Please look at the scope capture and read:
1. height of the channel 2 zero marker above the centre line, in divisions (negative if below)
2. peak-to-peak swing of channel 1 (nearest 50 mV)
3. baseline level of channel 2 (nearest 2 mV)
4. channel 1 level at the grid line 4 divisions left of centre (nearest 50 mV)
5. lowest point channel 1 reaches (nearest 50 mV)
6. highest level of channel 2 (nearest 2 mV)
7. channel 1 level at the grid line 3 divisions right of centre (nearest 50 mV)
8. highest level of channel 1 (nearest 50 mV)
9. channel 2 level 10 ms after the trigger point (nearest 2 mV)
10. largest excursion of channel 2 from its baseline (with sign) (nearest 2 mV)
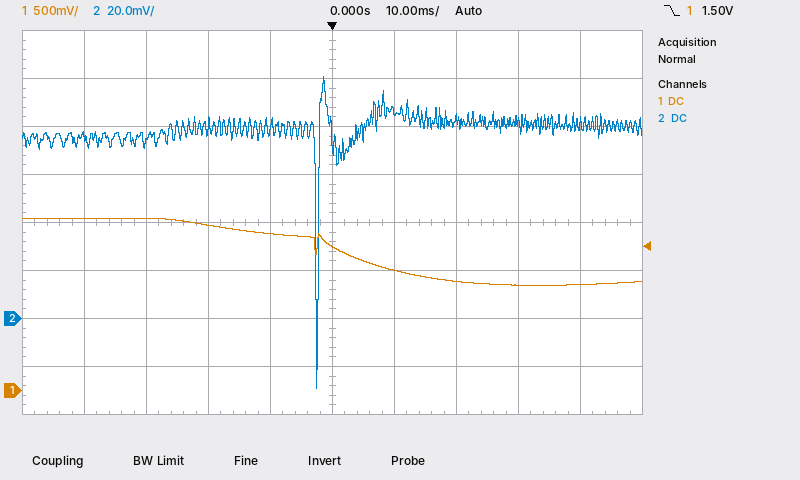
-2.0 div
700 mV
80 mV
1.80 V
1.10 V
100 mV
1.10 V
1.80 V
86 mV
-110 mV
